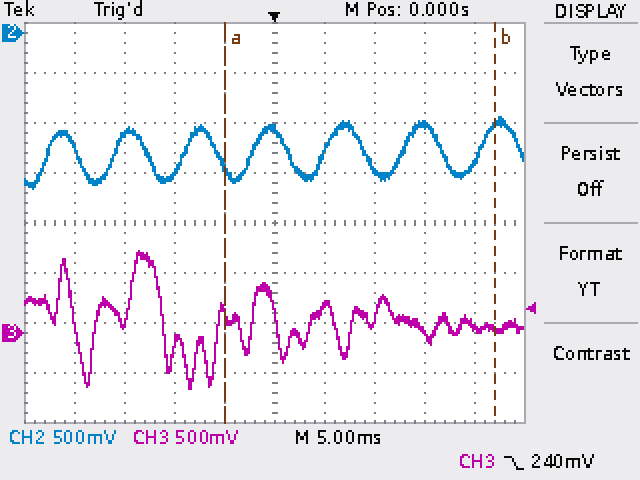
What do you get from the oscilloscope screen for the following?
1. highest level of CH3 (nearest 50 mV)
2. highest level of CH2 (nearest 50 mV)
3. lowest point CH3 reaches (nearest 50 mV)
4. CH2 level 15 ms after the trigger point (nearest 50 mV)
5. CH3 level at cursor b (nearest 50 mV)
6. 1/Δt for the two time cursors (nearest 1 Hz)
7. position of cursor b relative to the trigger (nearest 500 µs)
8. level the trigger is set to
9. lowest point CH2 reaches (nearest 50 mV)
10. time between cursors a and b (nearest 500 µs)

800 mV
-850 mV
-550 mV
-900 mV
50 mV
37 Hz
+22.0 ms
240 mV
-1.55 V
27.0 ms
